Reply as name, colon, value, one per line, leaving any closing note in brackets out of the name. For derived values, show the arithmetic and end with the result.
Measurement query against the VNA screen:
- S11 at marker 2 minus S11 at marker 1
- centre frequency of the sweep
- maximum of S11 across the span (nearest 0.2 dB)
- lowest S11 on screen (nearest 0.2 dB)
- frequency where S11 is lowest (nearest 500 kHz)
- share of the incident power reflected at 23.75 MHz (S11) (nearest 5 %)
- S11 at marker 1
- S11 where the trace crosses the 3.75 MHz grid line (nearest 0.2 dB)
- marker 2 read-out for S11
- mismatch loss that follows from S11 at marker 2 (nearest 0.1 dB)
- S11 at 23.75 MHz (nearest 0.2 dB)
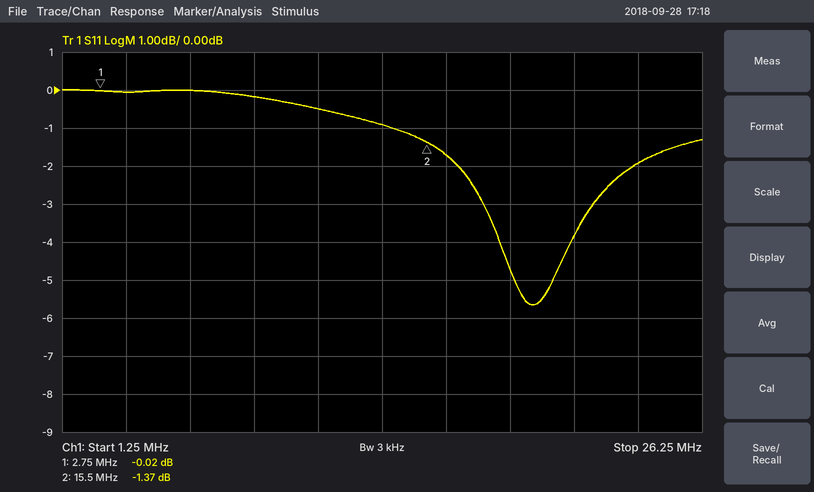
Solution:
S11 at marker 2 minus S11 at marker 1: -1.37 − (-0.02) = -1.35 dB
centre frequency of the sweep: 13.75 MHz
maximum of S11 across the span: 0.0 dB
lowest S11 on screen: -5.6 dB
frequency where S11 is lowest: 19.5 MHz
share of the incident power reflected at 23.75 MHz (S11): 10^(-2/10) ≈ 63.1 %, so 65 % to the nearest 5 %
S11 at marker 1: -0.02 dB
S11 where the trace crosses the 3.75 MHz grid line: 0.0 dB
marker 2 read-out for S11: -1.37 dB
mismatch loss that follows from S11 at marker 2: −10 log10(1 − 10^(-1.37/10)) ≈ 5.7 dB
S11 at 23.75 MHz: -2.0 dB
